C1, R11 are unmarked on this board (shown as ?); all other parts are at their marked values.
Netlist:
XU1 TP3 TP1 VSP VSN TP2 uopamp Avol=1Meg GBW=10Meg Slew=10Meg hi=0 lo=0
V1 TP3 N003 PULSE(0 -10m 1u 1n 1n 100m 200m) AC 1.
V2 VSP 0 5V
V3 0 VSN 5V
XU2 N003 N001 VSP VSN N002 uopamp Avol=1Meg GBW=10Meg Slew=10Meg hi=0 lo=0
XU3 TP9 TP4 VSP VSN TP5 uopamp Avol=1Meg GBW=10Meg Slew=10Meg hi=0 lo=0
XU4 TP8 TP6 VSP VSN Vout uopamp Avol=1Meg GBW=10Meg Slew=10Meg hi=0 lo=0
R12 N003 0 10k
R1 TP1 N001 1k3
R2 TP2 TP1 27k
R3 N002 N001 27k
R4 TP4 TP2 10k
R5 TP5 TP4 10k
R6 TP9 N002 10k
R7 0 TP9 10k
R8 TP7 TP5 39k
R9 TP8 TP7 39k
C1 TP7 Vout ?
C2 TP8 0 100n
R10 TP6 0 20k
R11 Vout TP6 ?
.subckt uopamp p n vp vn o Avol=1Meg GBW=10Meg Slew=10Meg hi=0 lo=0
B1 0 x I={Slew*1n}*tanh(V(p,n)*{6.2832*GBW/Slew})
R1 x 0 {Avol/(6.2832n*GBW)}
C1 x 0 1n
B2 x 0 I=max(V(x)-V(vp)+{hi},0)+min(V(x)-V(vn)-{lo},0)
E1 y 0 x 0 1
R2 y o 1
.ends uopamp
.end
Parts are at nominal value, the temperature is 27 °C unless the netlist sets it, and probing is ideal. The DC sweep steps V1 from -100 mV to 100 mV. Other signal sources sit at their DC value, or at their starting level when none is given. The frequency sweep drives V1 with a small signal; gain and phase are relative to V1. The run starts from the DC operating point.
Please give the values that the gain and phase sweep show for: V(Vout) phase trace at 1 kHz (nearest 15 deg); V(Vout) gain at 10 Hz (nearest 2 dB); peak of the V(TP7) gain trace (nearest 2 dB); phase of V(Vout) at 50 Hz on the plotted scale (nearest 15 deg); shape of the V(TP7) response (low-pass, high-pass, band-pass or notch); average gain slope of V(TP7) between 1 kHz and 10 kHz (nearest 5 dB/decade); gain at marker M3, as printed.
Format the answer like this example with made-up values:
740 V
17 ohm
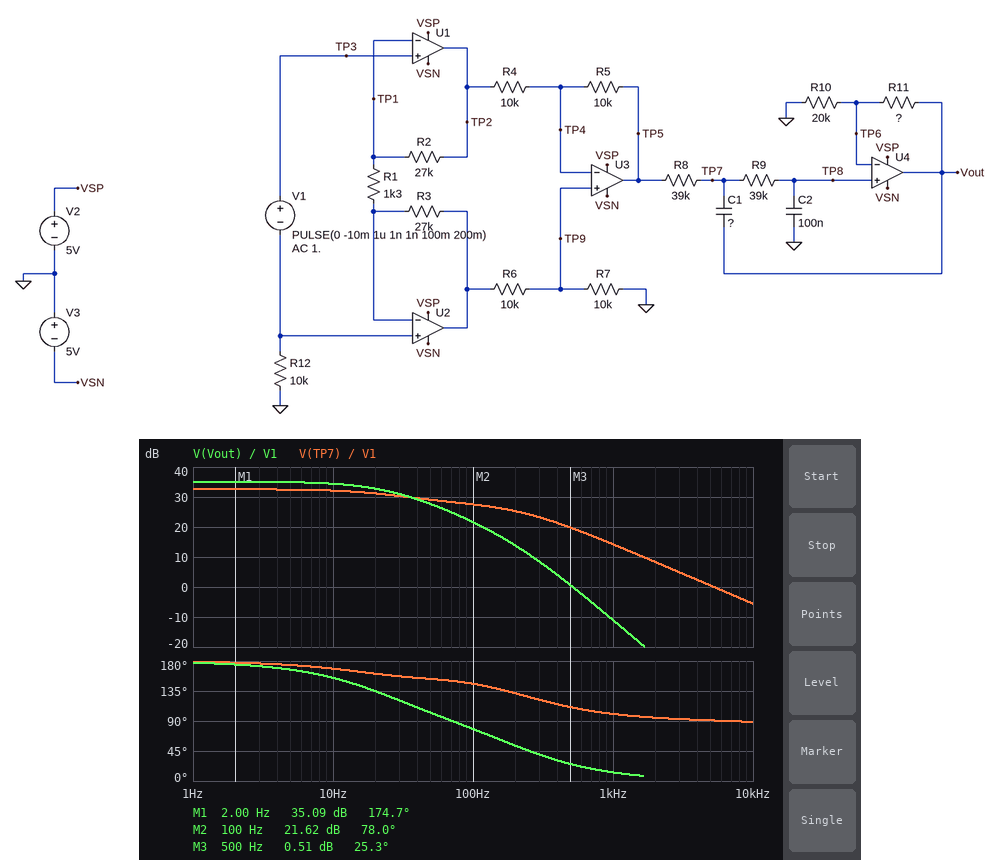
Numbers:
15 deg
34 dB
32 dB
105 deg
low-pass
-20 dB/decade
0.51 dB
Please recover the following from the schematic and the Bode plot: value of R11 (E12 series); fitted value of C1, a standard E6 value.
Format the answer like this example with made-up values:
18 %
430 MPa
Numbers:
6.8 kΩ
33 nF
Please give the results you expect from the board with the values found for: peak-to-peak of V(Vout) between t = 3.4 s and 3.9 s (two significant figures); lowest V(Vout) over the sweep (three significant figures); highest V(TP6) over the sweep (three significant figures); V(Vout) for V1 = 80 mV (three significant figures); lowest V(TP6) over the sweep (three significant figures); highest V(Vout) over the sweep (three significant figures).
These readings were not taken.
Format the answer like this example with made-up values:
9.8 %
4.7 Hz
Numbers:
570 mV
-5.01 V
3.74 V
-4.56 V
-3.74 V
5.01 V
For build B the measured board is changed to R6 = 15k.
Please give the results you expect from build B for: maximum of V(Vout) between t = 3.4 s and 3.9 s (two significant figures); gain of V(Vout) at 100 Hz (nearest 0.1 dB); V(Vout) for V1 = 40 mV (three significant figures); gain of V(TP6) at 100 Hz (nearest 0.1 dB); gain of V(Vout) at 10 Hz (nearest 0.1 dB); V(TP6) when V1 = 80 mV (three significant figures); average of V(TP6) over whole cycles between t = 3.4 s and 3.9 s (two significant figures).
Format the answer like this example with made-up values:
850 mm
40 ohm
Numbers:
510 mV
20.7 dB
-2.06 V
18.2 dB
33.5 dB
-3.07 V
190 mV
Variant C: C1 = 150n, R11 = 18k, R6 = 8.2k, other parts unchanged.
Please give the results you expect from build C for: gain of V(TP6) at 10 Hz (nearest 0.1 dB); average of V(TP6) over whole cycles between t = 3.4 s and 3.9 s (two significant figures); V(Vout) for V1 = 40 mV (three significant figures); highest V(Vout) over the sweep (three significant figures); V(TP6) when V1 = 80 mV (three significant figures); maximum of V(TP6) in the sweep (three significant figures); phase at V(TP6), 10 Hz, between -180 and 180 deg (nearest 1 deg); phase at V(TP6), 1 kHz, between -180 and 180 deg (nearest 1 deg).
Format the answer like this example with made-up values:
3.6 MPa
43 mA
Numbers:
33.7 dB
220 mV
-3.39 V
5.01 V
-2.64 V
2.64 V
170 deg
1 deg
